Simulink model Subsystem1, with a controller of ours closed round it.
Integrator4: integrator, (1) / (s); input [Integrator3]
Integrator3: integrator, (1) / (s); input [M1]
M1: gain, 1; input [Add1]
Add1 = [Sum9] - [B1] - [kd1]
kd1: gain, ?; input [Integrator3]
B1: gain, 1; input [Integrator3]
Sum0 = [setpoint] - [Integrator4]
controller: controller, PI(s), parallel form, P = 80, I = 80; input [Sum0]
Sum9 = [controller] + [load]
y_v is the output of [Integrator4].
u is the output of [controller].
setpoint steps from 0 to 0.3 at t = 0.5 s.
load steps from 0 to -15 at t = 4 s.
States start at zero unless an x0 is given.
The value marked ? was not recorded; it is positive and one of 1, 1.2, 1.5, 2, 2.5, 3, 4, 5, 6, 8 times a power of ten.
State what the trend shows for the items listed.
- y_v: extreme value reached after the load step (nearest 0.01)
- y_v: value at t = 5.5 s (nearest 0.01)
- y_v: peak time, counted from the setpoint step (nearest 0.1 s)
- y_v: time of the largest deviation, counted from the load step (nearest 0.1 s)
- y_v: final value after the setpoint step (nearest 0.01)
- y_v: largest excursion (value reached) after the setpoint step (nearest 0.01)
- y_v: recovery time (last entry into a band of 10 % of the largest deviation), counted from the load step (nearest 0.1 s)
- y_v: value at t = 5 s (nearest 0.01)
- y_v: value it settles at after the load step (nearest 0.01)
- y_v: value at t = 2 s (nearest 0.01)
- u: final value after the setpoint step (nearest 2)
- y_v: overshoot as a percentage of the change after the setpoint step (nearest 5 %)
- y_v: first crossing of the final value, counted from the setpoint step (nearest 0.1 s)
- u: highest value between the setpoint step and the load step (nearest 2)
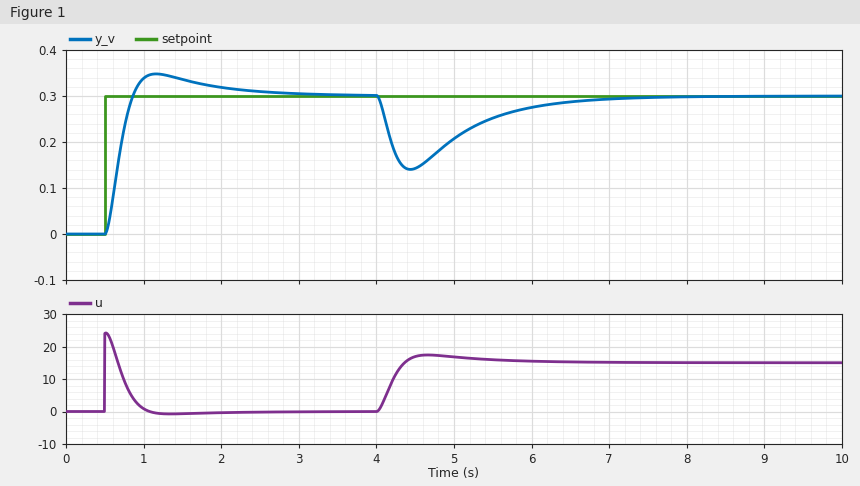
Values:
0.14
0.25
0.7 s
0.4 s
0.30
0.35
2.3 s
0.21
0.30
0.32
0
15 %
0.4 s
24
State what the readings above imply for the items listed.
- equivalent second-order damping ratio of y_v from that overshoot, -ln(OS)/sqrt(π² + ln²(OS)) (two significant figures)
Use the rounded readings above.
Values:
0.52
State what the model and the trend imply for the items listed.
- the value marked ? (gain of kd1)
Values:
15
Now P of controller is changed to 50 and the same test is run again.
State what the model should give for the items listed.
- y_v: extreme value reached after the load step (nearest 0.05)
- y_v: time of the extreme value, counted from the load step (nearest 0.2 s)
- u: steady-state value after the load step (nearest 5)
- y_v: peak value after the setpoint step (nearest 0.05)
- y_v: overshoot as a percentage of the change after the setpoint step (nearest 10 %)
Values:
0.10
0.6 s
15
0.40
30 %
